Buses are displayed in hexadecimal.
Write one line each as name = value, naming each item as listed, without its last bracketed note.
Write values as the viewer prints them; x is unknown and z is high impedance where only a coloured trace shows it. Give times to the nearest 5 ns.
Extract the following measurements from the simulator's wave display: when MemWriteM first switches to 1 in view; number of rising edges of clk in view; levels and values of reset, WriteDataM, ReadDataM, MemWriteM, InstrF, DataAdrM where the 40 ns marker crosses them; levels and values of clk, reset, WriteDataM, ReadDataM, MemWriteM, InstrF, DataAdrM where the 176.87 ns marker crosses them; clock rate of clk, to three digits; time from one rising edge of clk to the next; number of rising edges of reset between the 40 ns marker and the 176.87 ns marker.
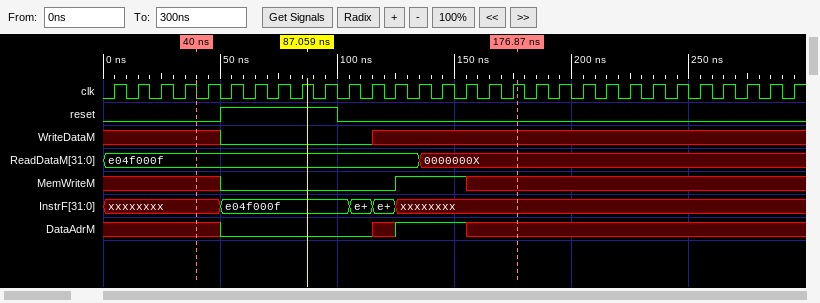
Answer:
when MemWriteM first switches to 1 in view = 125 ns
number of rising edges of clk in view = 30
levels and values of reset, WriteDataM, ReadDataM, MemWriteM, InstrF, DataAdrM where the 40 ns marker crosses them = reset=0, WriteDataM=x, ReadDataM=e04f000f, MemWriteM=x, InstrF=xxxxxxxx, DataAdrM=x
levels and values of clk, reset, WriteDataM, ReadDataM, MemWriteM, InstrF, DataAdrM where the 176.87 ns marker crosses them = clk=1, reset=0, WriteDataM=x, ReadDataM=0000000X, MemWriteM=x, InstrF=xxxxxxxx, DataAdrM=x
clock rate of clk, to three digits = 100 MHz
time from one rising edge of clk to the next = 10 ns
number of rising edges of reset between the 40 ns marker and the 176.87 ns marker = 1
